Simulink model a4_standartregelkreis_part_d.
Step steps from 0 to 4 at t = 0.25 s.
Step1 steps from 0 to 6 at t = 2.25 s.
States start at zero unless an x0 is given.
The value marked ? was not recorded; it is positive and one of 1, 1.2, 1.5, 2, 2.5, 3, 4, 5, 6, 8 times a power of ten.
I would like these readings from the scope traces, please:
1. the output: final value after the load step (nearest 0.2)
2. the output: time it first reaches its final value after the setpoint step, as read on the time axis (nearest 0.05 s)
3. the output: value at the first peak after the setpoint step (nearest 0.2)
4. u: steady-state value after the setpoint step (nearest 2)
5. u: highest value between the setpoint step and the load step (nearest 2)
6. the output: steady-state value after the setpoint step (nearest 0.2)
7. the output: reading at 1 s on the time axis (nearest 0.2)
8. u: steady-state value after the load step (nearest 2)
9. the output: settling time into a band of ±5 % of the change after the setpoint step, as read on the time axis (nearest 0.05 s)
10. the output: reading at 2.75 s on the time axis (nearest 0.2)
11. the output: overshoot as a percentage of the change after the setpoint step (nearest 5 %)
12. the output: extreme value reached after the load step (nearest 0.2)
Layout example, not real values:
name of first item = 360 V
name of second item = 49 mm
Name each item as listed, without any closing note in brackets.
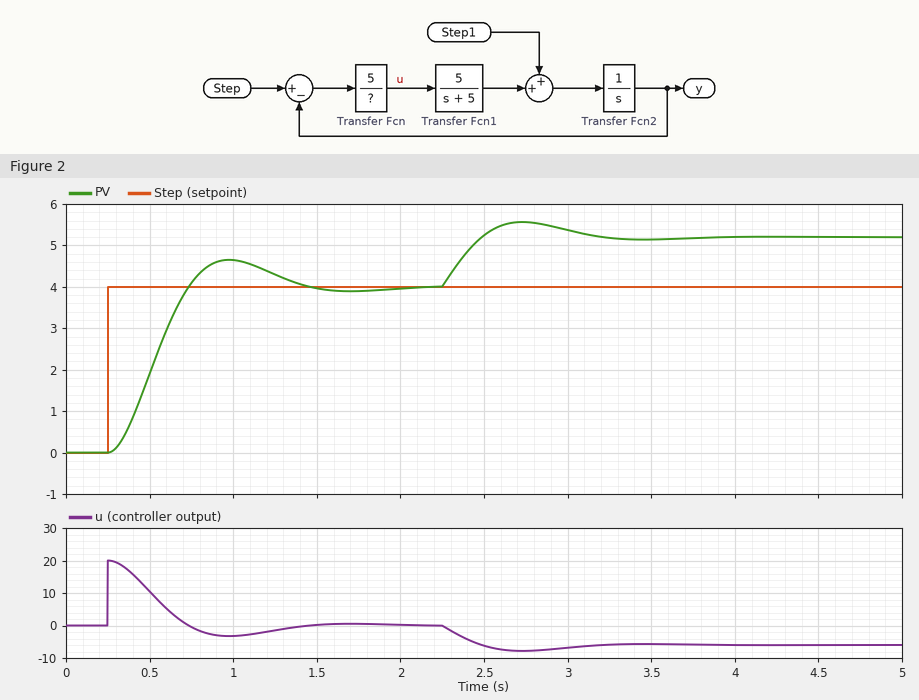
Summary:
the output: final value after the load step = 5.2
the output: time it first reaches its final value after the setpoint step, as read on the time axis = 0.75 s
the output: value at the first peak after the setpoint step = 4.6
u: steady-state value after the setpoint step = 0
u: highest value between the setpoint step and the load step = 20
the output: steady-state value after the setpoint step = 4.0
the output: reading at 1 s on the time axis = 4.6
u: steady-state value after the load step = -6
the output: settling time into a band of ±5 % of the change after the setpoint step, as read on the time axis = 1.30 s
the output: reading at 2.75 s on the time axis = 5.6
the output: overshoot as a percentage of the change after the setpoint step = 15 %
the output: extreme value reached after the load step = 5.6
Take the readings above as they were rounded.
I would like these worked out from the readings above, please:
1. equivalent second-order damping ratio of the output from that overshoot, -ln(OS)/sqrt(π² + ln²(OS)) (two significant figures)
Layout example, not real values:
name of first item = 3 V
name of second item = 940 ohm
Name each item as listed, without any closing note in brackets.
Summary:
equivalent second-order damping ratio of the output from that overshoot, -ln(OS)/sqrt(π² + ln²(OS)) = 0.52
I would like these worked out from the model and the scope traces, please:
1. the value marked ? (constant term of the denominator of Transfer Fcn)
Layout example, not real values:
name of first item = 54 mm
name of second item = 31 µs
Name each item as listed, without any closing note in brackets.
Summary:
the value marked ? = 1
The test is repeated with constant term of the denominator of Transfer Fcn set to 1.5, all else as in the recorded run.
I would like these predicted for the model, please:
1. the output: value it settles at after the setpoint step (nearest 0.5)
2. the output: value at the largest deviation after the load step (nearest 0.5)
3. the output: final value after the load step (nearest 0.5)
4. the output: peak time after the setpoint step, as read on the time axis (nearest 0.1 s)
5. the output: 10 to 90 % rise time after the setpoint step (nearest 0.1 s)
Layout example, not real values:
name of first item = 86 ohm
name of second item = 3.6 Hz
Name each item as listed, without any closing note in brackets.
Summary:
the output: value it settles at after the setpoint step = 4.0
the output: value at the largest deviation after the load step = 6.0
the output: final value after the load step = 6.0
the output: peak time after the setpoint step, as read on the time axis = 1.2 s
the output: 10 to 90 % rise time after the setpoint step = 0.5 s
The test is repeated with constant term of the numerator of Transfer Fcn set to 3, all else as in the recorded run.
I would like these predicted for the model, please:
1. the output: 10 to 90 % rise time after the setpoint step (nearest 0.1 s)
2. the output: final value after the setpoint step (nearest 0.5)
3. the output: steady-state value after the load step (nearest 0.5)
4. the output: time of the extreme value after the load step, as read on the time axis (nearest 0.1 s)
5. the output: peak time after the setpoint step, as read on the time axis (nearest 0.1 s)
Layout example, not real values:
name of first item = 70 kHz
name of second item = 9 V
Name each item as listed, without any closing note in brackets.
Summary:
the output: 10 to 90 % rise time after the setpoint step = 0.5 s
the output: final value after the setpoint step = 4.0
the output: steady-state value after the load step = 6.0
the output: time of the extreme value after the load step, as read on the time axis = 3.0 s
the output: peak time after the setpoint step, as read on the time axis = 1.3 s
